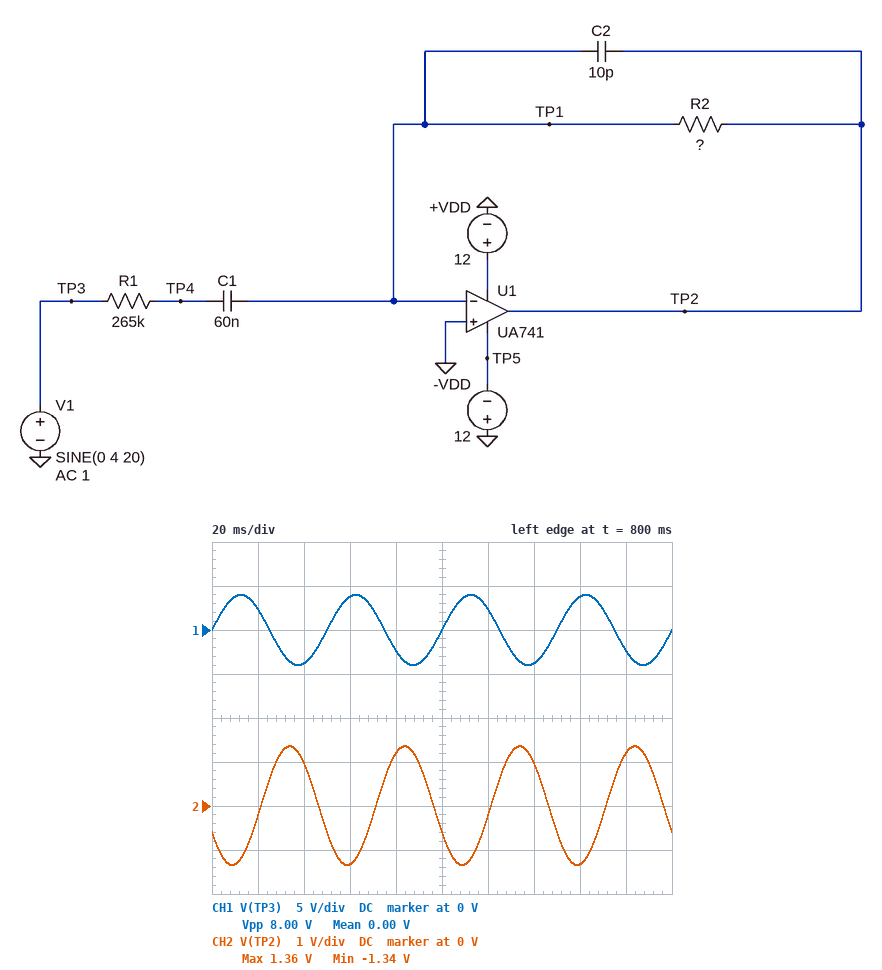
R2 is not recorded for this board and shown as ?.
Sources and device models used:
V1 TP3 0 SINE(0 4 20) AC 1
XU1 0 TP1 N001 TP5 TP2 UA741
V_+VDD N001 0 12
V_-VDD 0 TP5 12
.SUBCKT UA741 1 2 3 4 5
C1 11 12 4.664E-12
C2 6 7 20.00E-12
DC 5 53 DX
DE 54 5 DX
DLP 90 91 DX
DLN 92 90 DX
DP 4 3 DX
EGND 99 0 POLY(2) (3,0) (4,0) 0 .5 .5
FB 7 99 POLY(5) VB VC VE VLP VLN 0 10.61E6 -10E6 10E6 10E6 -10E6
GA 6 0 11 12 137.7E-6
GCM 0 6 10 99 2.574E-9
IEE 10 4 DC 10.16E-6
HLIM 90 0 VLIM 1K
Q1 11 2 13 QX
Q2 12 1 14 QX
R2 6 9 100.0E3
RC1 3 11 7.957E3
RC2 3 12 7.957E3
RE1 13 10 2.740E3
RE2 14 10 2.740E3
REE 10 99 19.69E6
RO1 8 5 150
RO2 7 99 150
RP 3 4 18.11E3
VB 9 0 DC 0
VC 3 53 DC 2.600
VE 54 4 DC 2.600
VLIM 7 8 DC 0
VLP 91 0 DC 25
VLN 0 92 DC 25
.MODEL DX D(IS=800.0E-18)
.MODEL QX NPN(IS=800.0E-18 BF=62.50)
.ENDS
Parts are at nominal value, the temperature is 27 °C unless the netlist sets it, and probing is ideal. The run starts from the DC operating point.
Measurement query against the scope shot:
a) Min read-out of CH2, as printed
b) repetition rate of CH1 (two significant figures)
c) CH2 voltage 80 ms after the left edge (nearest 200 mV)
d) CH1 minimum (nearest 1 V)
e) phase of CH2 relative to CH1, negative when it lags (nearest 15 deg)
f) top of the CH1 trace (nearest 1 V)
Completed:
-1.34 V
20 Hz
1.2 V
-4 V
-150 deg
4 V
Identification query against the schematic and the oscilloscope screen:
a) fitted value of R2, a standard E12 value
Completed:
100 kΩ
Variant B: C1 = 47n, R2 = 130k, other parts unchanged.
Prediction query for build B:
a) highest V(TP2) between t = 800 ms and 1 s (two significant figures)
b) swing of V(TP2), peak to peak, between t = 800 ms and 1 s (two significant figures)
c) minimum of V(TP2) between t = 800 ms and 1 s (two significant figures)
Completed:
1.7 V
3.3 V
-1.6 V
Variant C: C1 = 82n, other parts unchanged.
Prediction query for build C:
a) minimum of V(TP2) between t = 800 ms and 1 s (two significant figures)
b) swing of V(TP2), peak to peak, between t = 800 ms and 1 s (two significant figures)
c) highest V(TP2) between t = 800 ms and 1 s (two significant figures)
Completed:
-1.4 V
2.8 V
1.4 V
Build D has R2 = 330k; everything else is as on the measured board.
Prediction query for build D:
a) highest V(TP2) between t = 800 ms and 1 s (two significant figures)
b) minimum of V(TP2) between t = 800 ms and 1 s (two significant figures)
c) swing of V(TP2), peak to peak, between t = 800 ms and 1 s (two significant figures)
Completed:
4.5 V
-4.4 V
8.9 V
